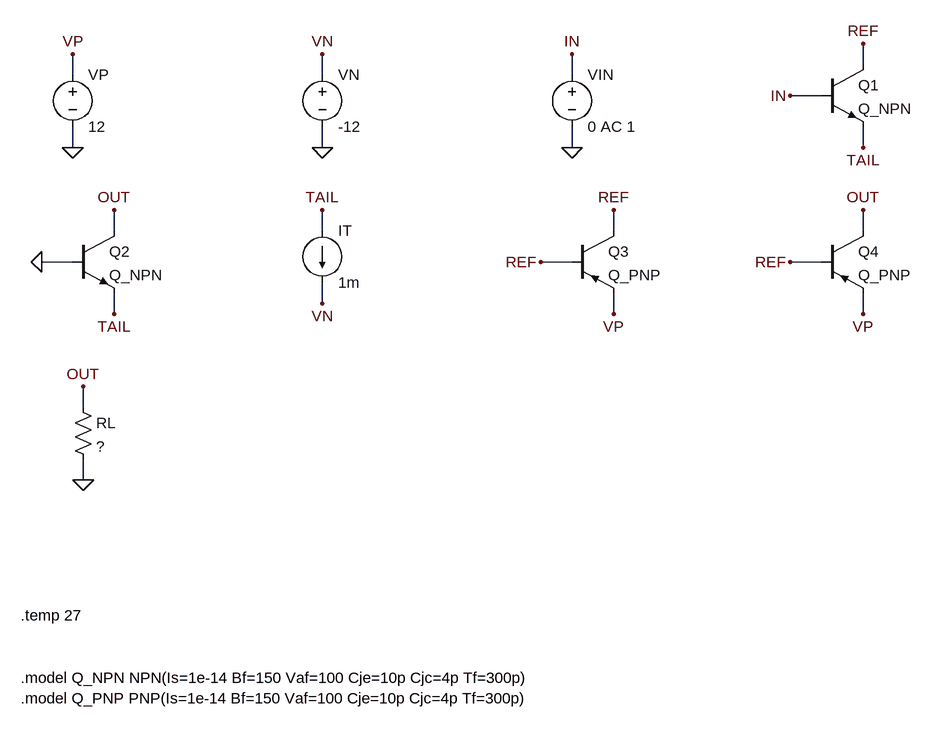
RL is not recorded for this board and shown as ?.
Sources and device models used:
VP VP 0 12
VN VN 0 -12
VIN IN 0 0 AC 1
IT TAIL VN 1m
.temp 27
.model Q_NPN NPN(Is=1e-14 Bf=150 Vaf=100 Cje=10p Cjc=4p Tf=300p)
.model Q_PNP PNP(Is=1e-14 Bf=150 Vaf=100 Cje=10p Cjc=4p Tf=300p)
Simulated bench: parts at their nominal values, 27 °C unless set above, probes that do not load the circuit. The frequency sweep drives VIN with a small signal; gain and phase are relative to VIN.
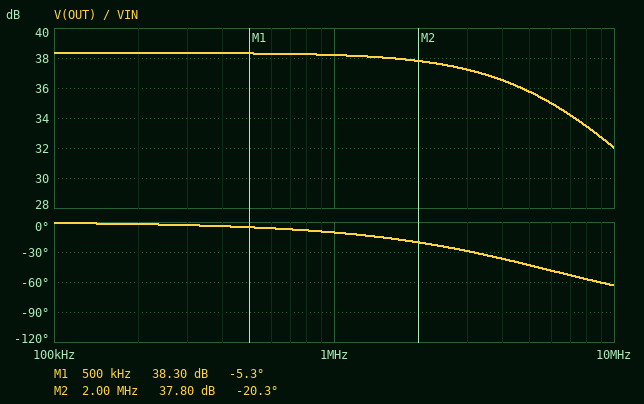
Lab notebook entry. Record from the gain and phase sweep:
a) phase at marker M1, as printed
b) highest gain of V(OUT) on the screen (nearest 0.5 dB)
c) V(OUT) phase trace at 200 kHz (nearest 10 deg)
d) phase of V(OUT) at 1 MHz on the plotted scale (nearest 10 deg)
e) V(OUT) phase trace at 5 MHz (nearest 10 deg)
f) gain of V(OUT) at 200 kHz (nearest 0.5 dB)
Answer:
-5.3 deg
38.5 dB
0 deg
-10 deg
-40 deg
38.5 dB
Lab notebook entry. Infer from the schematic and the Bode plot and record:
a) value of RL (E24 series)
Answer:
4.3 kΩ
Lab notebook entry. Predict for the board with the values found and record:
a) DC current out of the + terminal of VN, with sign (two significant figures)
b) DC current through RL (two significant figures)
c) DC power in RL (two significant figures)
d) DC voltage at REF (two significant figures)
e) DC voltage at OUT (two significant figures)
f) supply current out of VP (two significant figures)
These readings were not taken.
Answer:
-1.0 mA
100 µA
44 µW
11 V
430 mV
1.1 mA
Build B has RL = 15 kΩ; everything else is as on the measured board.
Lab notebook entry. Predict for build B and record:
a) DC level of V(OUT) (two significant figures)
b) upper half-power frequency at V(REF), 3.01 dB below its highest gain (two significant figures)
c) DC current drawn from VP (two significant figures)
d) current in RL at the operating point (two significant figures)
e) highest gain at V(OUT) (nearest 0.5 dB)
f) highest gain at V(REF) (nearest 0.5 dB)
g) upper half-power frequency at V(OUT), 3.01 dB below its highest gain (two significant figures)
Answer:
1.4 V
2.6 MHz
1.1 mA
91 µA
48.5 dB
-7.0 dB
1.9 MHz
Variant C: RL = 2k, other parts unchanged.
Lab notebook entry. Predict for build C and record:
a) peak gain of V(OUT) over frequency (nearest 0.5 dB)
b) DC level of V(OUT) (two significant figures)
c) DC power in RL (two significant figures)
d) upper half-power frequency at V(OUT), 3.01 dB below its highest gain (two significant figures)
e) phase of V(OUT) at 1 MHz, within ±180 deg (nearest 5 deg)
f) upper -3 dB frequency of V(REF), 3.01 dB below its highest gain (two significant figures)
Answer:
32.0 dB
210 mV
21 µW
11 MHz
-5 deg
15 MHz
